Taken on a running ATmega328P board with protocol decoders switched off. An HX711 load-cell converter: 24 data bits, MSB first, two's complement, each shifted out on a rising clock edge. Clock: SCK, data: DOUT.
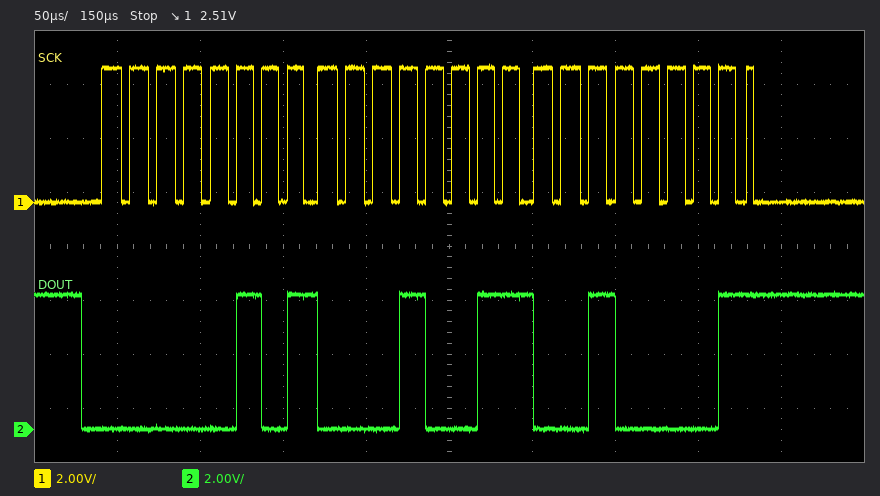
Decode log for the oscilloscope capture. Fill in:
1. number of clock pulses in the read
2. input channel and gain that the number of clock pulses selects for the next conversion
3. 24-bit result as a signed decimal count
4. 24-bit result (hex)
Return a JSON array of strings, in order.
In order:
["25", "channel A, gain 128", "332577", "0x051321"]
